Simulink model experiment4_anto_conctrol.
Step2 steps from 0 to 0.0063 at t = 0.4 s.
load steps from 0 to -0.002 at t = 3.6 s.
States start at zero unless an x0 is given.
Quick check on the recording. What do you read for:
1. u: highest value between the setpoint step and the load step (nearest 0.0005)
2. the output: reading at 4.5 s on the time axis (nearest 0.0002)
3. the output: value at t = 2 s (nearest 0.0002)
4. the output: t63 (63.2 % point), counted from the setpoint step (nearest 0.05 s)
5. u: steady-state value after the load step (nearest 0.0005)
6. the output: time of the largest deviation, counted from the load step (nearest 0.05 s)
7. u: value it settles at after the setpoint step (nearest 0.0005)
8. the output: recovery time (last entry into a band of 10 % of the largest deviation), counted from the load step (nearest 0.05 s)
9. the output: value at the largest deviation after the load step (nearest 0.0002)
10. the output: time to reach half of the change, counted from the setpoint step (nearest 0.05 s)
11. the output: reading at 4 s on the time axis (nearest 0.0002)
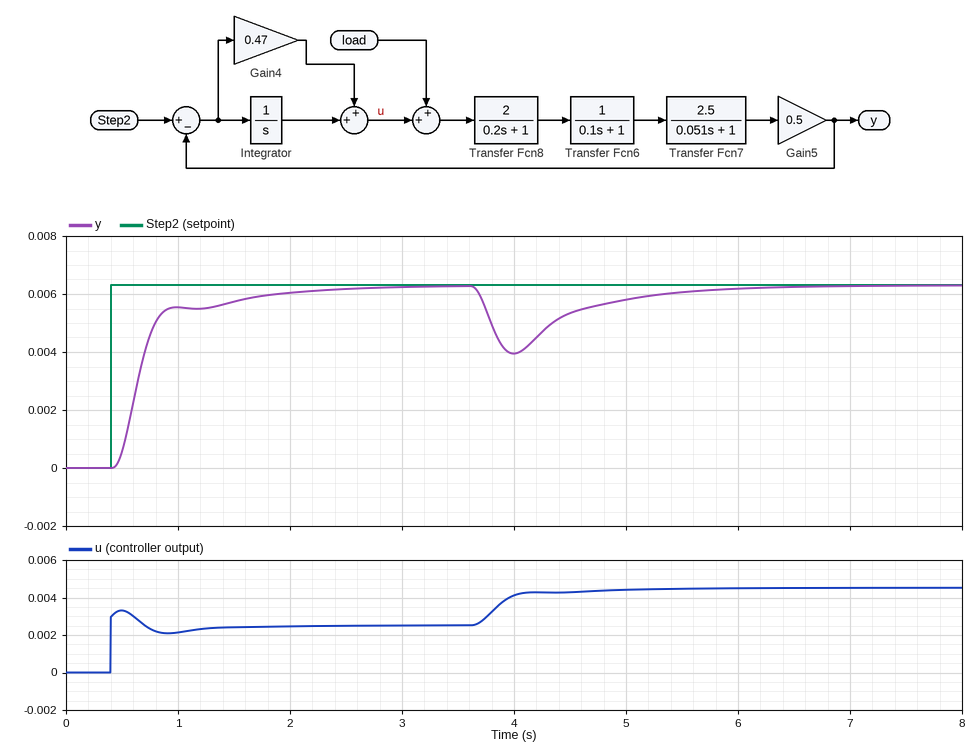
0.0035
0.0054
0.0060
0.30 s
0.0045
0.40 s
0.0025
1.90 s
0.0040
0.25 s
0.0040
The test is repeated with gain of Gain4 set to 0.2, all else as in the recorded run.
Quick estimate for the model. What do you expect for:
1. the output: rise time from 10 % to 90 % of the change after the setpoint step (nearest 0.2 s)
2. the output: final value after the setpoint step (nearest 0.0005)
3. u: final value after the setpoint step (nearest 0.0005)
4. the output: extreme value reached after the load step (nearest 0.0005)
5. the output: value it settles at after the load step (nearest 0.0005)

0.6 s
0.0065
0.0025
0.0035
0.0065
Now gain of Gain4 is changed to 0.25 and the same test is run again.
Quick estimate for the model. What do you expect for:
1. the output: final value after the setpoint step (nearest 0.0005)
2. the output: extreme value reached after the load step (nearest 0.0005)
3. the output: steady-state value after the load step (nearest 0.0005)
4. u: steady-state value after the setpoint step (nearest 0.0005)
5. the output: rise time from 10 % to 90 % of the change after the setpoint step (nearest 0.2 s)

0.0065
0.0035
0.0065
0.0025
0.6 s
